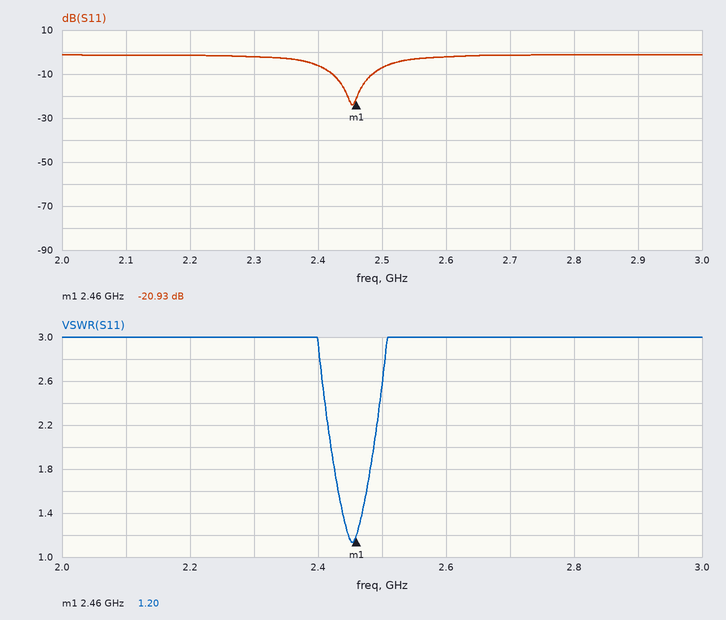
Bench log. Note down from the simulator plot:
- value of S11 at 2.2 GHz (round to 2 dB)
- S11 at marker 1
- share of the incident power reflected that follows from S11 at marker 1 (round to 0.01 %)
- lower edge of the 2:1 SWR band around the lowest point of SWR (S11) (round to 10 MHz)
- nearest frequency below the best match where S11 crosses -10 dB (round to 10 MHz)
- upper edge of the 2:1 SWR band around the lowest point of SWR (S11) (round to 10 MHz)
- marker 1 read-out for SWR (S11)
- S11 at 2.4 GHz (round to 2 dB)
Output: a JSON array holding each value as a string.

["-2 dB", "-20.93 dB", "0.81 %", "2.42 GHz", "2.42 GHz", "2.49 GHz", "1.20", "-6 dB"]
